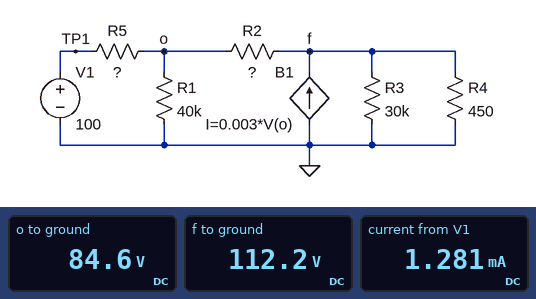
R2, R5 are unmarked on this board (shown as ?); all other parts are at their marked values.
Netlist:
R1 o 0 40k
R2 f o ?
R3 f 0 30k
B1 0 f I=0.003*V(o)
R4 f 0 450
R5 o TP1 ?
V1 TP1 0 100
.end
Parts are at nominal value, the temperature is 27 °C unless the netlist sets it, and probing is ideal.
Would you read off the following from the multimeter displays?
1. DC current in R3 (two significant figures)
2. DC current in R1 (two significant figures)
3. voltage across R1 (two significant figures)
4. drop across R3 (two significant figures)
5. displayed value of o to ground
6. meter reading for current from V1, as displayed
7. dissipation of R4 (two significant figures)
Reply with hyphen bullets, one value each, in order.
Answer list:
- 3.7 mA
- 2.1 mA
- 85 V
- 110 V
- 84.6 V
- 1.281 mA
- 28 W
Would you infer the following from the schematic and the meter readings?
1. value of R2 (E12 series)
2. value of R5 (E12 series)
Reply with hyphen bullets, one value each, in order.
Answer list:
- 33 kΩ
- 12 kΩ
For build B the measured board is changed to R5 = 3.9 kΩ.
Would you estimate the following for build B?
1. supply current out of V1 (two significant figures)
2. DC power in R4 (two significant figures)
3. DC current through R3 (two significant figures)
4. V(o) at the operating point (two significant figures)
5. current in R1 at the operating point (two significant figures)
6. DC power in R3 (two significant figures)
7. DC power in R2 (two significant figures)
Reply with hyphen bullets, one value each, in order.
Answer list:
- 1.4 mA
- 35 W
- 4.2 mA
- 94 V
- 2.4 mA
- 520 mW
- 29 mW
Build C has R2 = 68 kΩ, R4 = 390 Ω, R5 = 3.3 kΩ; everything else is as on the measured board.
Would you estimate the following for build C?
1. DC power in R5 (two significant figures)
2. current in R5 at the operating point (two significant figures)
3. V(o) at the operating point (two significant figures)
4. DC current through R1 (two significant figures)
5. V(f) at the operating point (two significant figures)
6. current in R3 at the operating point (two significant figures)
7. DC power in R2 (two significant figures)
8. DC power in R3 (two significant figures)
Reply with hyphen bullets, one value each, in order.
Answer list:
- 15 mW
- 2.1 mA
- 93 V
- 2.3 mA
- 110 V
- 3.6 mA
- 3.0 mW
- 380 mW
